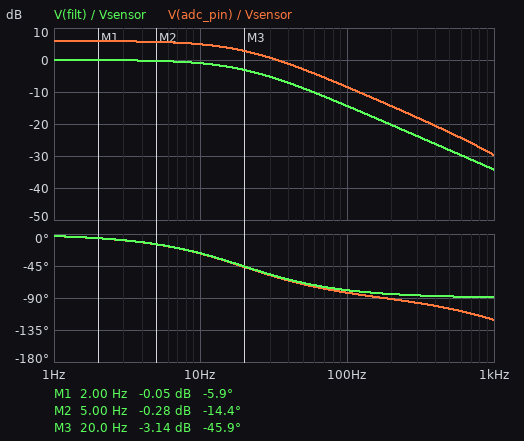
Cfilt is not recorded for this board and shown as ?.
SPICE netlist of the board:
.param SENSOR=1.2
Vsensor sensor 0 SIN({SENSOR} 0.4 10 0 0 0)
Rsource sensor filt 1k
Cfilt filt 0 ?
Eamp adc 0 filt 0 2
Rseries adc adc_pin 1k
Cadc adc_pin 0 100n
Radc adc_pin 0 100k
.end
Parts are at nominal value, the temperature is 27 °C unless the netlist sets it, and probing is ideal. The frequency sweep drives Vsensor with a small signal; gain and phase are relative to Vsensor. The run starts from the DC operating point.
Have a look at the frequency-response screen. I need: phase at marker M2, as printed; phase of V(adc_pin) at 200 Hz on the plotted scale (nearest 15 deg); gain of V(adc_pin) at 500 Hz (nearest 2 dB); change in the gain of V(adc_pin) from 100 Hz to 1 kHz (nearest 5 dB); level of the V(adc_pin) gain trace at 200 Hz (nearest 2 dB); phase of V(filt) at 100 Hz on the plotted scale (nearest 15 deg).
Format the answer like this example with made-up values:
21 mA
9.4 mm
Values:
-14.4 deg
-90 deg
-22 dB
-20 dB
-14 dB
-75 deg
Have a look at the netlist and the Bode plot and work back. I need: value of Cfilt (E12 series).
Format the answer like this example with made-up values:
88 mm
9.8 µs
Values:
8.2 µF
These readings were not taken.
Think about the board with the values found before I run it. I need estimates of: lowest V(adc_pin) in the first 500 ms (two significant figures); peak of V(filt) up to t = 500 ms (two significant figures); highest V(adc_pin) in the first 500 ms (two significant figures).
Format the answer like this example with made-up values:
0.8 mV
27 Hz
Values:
1.7 V
1.6 V
3.1 V
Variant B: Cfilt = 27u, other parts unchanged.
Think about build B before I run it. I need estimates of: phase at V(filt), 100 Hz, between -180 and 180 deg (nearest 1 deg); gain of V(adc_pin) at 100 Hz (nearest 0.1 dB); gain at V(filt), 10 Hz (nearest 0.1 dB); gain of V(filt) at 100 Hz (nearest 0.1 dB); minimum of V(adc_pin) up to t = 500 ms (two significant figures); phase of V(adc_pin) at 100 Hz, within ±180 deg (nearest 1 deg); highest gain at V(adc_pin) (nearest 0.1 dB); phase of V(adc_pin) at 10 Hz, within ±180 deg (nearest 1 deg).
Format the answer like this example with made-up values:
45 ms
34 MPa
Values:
-87 deg
-18.7 dB
-5.9 dB
-24.6 dB
2.0 V
-90 deg
5.9 dB
-60 deg
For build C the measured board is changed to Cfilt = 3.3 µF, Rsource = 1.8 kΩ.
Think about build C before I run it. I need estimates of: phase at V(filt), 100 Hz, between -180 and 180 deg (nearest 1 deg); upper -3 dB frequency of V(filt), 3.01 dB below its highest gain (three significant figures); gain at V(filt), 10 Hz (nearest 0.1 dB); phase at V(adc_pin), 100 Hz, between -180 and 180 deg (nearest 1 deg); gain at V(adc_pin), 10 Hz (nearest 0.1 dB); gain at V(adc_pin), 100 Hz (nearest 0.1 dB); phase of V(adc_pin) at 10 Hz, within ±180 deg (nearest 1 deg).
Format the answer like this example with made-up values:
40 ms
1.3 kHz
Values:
-75 deg
26.8 Hz
-0.6 dB
-79 deg
5.4 dB
-5.8 dB
-21 deg
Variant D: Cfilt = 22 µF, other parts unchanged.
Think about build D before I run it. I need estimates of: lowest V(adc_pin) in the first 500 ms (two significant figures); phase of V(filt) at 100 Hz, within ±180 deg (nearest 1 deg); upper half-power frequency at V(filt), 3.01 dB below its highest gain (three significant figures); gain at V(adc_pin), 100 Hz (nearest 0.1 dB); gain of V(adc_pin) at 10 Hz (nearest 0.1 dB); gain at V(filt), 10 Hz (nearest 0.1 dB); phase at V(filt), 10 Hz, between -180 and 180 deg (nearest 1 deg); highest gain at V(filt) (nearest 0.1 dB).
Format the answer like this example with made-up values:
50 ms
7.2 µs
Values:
1.9 V
-86 deg
7.23 Hz
-16.9 dB
1.3 dB
-4.6 dB
-54 deg
0 dB
